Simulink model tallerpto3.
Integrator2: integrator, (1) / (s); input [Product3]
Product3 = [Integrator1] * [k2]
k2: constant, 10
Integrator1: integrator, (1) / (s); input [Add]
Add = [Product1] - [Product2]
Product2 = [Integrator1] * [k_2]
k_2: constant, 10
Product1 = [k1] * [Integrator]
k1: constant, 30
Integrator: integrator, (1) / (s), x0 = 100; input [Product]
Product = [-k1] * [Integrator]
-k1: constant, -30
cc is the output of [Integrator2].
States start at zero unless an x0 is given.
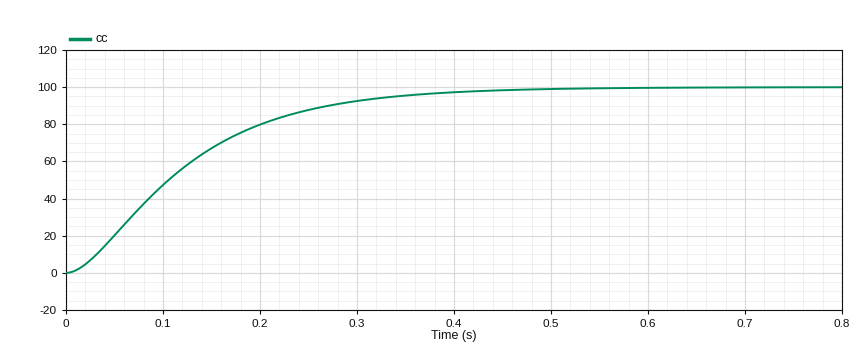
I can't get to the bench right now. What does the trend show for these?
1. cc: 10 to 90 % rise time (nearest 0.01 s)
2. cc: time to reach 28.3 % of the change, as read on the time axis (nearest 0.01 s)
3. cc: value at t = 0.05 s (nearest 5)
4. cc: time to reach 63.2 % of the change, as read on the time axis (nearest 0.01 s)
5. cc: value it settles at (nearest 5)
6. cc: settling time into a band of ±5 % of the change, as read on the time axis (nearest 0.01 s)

0.24 s
0.06 s
20
0.14 s
100
0.34 s
